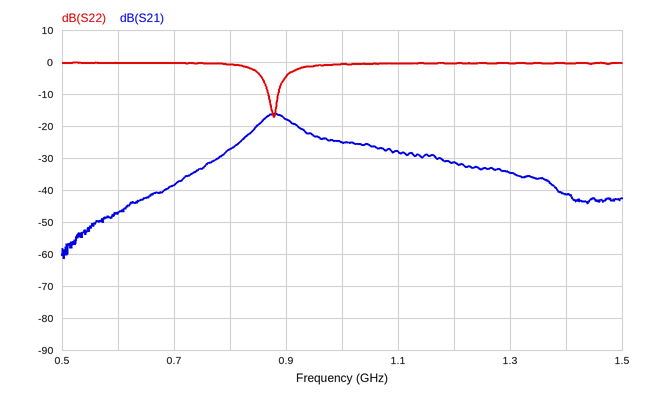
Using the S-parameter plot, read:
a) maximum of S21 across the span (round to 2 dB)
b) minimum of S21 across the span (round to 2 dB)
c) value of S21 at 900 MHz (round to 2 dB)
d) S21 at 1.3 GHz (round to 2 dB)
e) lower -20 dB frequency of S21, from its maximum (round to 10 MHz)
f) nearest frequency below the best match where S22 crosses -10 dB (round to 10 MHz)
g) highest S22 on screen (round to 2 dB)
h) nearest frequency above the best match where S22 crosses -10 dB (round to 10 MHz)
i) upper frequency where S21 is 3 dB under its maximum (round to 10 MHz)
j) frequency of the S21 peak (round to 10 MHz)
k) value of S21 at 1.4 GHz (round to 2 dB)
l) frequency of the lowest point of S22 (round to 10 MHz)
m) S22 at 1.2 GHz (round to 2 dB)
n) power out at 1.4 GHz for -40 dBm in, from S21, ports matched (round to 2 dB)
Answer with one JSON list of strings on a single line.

["-16 dB", "-62 dB", "-18 dB", "-34 dB", "720 MHz", "870 MHz", "0 dB", "890 MHz", "910 MHz", "880 MHz", "-42 dB", "880 MHz", "0 dB", "-82 dBm"]
